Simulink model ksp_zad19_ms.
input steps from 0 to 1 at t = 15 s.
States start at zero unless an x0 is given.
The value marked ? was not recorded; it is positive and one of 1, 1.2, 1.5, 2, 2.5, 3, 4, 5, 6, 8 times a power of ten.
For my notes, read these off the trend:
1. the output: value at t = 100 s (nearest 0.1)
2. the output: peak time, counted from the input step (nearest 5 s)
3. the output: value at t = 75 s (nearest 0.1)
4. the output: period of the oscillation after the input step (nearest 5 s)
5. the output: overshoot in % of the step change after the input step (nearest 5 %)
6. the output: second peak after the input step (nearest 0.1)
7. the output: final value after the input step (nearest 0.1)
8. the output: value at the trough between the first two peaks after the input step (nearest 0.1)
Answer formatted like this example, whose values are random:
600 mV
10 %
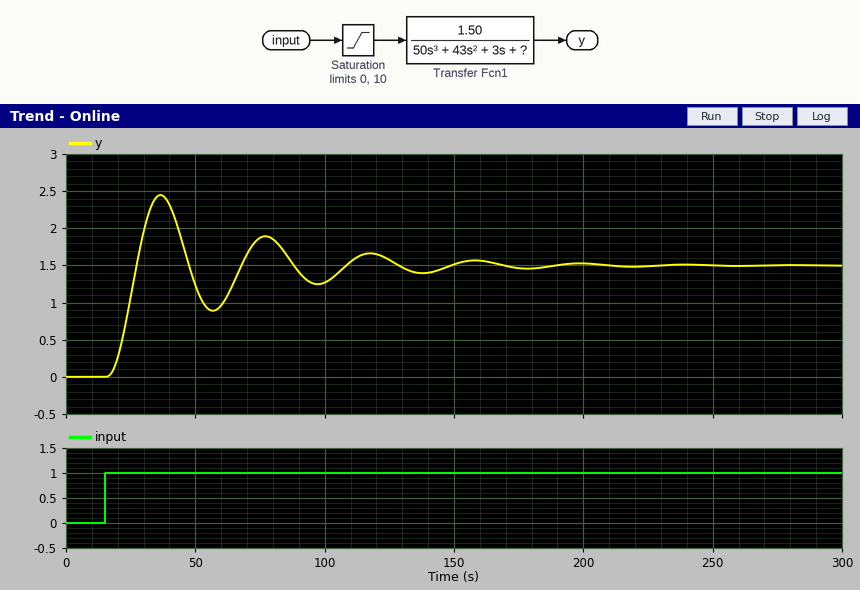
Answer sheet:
1.3
20 s
1.9
40 s
65 %
1.9
1.5
0.9
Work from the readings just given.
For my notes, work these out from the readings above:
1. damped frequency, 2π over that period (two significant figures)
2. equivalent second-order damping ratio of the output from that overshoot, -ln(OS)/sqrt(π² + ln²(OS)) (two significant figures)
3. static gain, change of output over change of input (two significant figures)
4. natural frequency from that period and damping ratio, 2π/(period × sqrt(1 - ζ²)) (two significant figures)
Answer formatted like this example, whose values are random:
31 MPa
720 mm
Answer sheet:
0.16 rad/s
0.14
1.5
0.16 rad/s
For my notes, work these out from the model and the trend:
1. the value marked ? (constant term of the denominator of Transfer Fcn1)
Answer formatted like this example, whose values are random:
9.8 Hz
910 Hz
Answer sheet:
1
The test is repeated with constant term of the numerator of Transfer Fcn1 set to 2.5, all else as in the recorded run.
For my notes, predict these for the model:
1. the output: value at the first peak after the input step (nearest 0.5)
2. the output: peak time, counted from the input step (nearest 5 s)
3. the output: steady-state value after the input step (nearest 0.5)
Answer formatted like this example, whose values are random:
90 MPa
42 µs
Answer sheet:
4.0
20 s
2.5
